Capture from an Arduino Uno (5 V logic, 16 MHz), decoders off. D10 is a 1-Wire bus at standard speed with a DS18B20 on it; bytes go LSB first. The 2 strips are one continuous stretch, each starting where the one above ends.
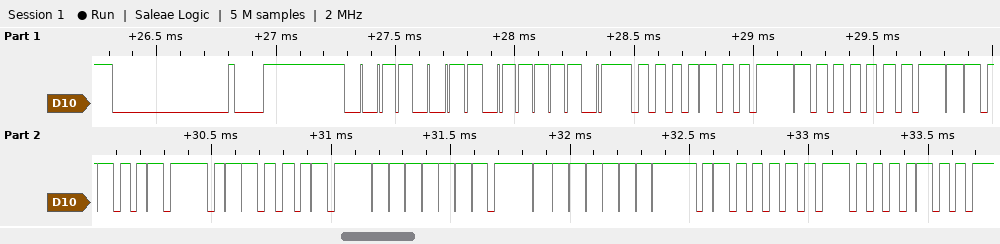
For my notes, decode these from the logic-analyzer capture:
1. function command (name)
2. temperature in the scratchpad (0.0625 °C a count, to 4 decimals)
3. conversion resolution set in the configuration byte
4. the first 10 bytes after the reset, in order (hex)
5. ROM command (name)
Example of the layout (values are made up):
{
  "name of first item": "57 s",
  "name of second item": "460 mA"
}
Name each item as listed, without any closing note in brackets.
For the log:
{
  "function command": "Read Scratchpad",
  "temperature in the scratchpad": "17.0000 °C",
  "conversion resolution set in the configuration byte": "12 bits",
  "the first 10 bytes after the reset, in order": "CC BE 10 01 4B 46 7F FF 02 10",
  "ROM command": "Skip ROM"
}
